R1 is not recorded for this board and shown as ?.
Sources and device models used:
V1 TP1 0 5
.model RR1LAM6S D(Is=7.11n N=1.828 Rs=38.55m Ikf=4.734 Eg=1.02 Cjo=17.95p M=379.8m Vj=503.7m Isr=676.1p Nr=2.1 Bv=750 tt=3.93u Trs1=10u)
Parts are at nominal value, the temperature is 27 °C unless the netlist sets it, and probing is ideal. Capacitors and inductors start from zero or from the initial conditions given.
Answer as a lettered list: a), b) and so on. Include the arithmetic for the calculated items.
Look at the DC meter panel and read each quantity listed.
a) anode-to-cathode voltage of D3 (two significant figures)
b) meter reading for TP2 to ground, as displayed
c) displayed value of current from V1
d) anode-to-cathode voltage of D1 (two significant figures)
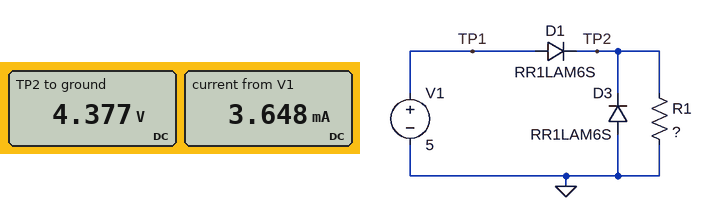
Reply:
a) 0 V - 4.377 V = -4.4 V
b) 4.377 V
c) 3.648 mA
d) 5 V - 4.377 V = 620 mV
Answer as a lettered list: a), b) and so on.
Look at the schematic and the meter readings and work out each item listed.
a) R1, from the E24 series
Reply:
a) 1.2 kΩ
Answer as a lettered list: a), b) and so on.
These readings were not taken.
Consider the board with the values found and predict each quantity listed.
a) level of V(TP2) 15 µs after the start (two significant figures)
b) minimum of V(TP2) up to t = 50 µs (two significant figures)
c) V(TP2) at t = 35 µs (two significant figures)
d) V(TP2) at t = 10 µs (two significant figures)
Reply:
a) 4.4 V
b) 4.4 V
c) 4.4 V
d) 4.4 V
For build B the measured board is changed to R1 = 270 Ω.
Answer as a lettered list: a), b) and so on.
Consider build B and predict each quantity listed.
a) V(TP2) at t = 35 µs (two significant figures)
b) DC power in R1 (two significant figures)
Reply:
a) 4.3 V
b) 69 mW
